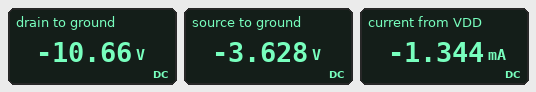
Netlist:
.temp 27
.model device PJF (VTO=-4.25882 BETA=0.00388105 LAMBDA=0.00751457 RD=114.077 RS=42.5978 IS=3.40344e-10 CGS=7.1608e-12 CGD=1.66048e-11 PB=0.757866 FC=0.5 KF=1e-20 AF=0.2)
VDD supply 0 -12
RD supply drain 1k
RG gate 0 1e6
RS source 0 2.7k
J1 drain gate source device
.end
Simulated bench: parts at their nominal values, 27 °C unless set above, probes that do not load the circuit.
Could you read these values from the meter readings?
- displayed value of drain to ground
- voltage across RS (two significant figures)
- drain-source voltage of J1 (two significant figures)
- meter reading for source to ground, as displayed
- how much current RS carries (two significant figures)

-10.66 V
3.6 V
-7.0 V
-3.628 V
1.3 mA
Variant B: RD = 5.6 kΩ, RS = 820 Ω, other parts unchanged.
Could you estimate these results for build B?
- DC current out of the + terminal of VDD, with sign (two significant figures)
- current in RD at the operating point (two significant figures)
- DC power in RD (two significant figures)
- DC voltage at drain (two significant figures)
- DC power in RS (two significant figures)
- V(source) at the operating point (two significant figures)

-1.8 mA
1.8 mA
18 mW
-1.9 V
2.7 mW
-1.5 V
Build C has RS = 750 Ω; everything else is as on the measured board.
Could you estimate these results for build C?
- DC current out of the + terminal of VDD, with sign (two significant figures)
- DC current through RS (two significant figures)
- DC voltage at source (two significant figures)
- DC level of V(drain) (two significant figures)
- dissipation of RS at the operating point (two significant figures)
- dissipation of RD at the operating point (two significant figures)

-4.1 mA
4.1 mA
-3.1 V
-7.9 V
13 mW
17 mW
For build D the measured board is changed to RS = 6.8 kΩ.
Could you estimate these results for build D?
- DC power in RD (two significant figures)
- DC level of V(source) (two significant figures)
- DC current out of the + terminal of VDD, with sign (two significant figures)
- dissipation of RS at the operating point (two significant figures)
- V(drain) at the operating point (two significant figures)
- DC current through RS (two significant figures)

320 µW
-3.9 V
-570 µA
2.2 mW
-11 V
570 µA
